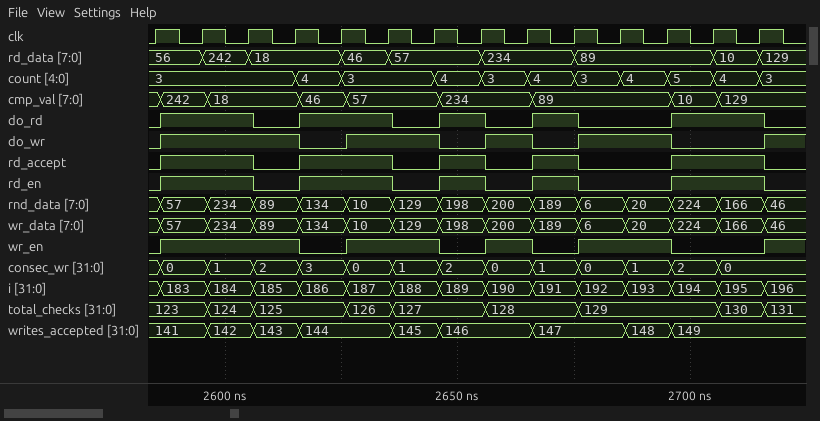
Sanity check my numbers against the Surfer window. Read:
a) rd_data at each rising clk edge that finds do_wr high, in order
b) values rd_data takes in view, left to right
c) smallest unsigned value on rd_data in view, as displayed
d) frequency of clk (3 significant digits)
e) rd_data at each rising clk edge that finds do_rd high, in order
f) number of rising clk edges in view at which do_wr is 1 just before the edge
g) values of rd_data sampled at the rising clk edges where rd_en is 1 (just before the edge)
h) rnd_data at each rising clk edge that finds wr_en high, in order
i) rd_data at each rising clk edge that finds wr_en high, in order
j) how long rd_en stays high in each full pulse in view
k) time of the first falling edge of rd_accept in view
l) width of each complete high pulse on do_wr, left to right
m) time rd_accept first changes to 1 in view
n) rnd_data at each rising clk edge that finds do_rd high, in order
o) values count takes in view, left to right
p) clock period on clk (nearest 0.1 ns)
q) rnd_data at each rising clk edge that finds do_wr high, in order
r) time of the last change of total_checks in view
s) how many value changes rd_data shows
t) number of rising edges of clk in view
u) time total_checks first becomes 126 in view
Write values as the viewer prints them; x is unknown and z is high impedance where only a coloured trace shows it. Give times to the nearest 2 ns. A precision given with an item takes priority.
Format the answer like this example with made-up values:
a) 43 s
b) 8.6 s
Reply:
a) 56, 242, 18, 46, 57, 234, 89, 89
b) 56, 242, 18, 46, 57, 234, 89, 10, 129
c) 10
d) 100 MHz
e) 56, 242, 18, 46, 57, 234, 89, 10
f) 8
g) 56, 242, 18, 46, 57, 234, 89, 10
h) 57, 234, 89, 10, 129, 200, 6, 20
i) 56, 242, 18, 46, 57, 234, 89, 89
j) 20 ns, 20 ns, 10 ns, 10 ns, 20 ns
k) 2606 ns
l) 30 ns, 20 ns, 10 ns, 20 ns
m) 2586 ns
n) 57, 234, 134, 10, 198, 189, 224, 166
o) 3, 4, 3, 4, 3, 4, 3, 4, 5, 4, 3
p) 10 ns
q) 57, 234, 89, 10, 129, 200, 6, 20
r) 2716 ns
s) 8
t) 14
u) 2626 ns
